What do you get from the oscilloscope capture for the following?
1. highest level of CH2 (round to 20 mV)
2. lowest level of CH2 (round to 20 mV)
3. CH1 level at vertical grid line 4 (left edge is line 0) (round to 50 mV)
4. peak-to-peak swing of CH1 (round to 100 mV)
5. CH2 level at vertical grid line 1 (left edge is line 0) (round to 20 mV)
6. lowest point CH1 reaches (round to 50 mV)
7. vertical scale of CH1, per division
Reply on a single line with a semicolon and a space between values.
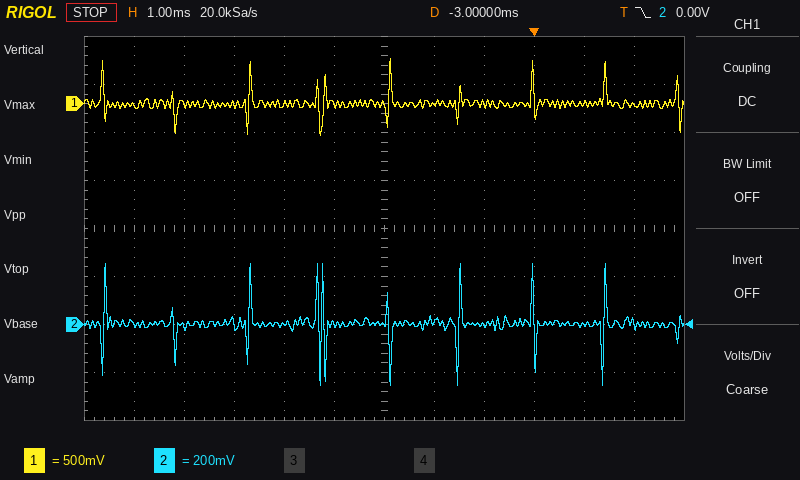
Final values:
260 mV; -260 mV; 0 mV; 800 mV; 0 mV; -350 mV; 500 mV
